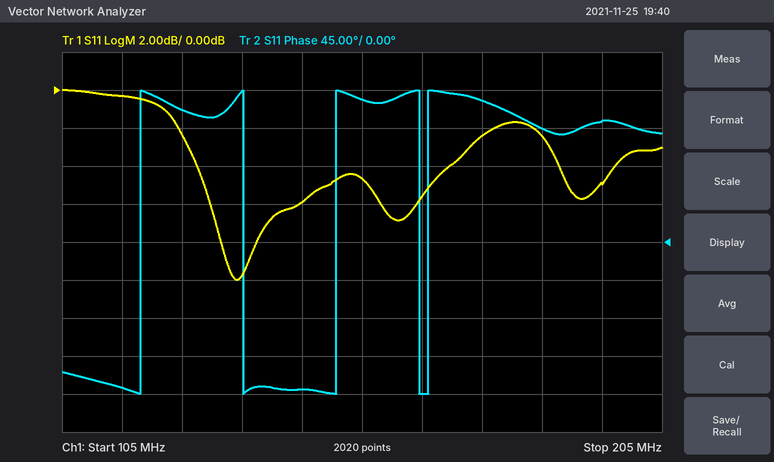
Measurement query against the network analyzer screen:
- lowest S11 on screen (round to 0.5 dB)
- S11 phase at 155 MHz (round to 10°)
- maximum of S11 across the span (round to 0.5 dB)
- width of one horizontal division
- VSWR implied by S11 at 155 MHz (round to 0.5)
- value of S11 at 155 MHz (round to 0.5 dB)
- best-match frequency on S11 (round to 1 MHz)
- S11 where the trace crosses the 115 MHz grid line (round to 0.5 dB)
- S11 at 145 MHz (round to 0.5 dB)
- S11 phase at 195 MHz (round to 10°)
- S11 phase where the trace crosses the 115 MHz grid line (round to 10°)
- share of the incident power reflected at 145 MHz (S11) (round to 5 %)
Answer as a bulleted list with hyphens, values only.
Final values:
- -10.0 dB
- 170°
- 0.0 dB
- 10 MHz
- 4.0
- -4.5 dB
- 134 MHz
- -0.5 dB
- -6.0 dB
- 140°
- -170°
- 25 %
